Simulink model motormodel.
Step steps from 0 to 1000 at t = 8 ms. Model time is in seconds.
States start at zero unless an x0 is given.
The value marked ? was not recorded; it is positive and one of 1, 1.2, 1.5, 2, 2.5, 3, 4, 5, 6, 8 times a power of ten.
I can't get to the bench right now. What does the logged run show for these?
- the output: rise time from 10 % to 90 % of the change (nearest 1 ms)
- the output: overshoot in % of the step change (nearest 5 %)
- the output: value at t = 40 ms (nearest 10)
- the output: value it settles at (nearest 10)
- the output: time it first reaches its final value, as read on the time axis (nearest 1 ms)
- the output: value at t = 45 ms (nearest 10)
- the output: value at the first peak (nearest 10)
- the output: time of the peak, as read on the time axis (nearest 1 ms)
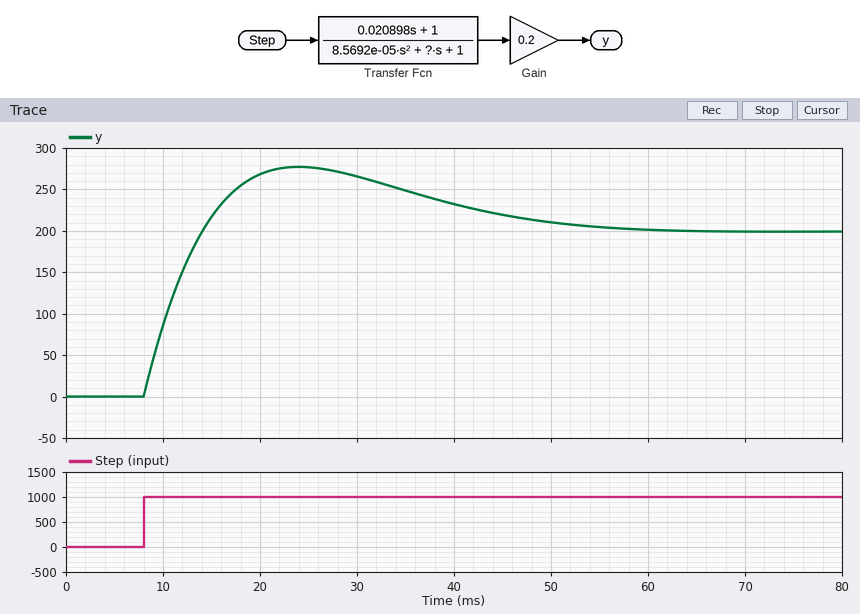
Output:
5 ms
40 %
230
200
14 ms
220
280
24 ms
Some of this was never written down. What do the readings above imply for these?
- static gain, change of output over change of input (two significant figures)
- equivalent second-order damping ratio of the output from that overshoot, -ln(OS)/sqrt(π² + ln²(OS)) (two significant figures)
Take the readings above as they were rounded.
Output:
0.20
0.28
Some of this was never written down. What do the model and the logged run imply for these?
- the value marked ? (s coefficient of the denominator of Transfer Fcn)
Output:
0.015
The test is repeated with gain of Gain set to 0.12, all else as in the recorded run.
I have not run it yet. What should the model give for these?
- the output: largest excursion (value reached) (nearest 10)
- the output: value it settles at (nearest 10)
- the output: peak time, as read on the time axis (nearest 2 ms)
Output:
170
120
24 ms
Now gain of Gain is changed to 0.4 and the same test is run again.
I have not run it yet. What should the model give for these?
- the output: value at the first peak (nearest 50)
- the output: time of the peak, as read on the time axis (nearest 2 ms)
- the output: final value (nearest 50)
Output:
550
24 ms
400
